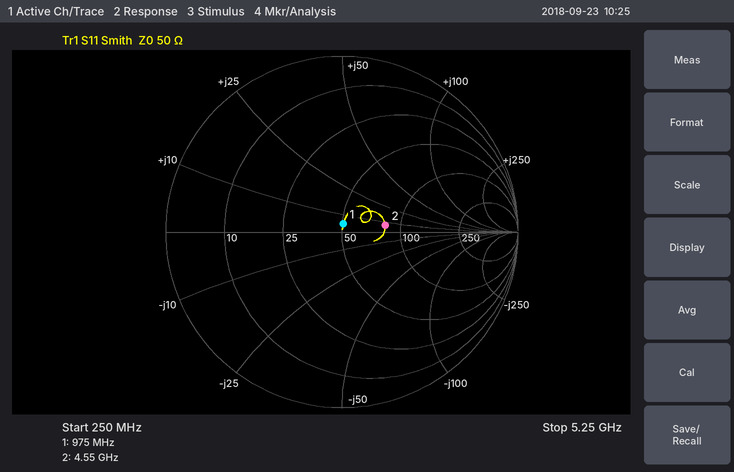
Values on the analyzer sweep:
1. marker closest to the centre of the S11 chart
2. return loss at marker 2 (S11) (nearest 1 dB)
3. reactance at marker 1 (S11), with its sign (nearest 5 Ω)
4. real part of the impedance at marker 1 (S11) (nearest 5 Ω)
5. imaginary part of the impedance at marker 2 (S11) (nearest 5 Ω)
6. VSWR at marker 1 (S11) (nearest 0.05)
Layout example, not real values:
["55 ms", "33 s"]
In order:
["marker 1", "12 dB", "+5 Ω", "50 Ω", "+5 Ω", "1.10"]
